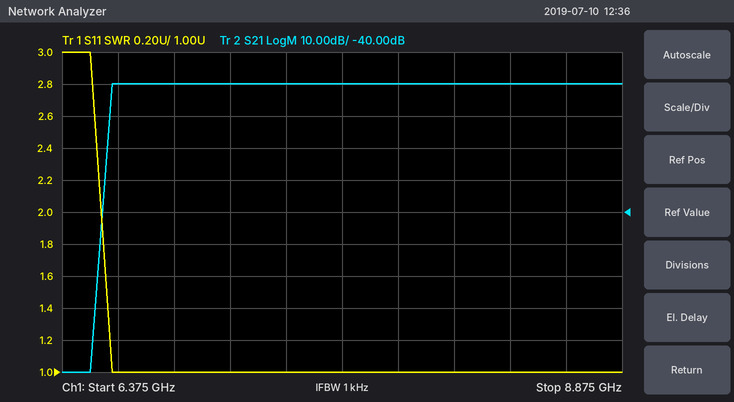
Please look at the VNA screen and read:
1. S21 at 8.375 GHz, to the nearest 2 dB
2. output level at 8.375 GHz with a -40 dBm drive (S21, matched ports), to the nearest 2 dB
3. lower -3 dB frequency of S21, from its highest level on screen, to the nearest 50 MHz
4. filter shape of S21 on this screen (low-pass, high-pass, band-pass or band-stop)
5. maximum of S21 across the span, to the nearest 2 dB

0 dB
-40 dBm
6.60 GHz
high-pass
0 dB
